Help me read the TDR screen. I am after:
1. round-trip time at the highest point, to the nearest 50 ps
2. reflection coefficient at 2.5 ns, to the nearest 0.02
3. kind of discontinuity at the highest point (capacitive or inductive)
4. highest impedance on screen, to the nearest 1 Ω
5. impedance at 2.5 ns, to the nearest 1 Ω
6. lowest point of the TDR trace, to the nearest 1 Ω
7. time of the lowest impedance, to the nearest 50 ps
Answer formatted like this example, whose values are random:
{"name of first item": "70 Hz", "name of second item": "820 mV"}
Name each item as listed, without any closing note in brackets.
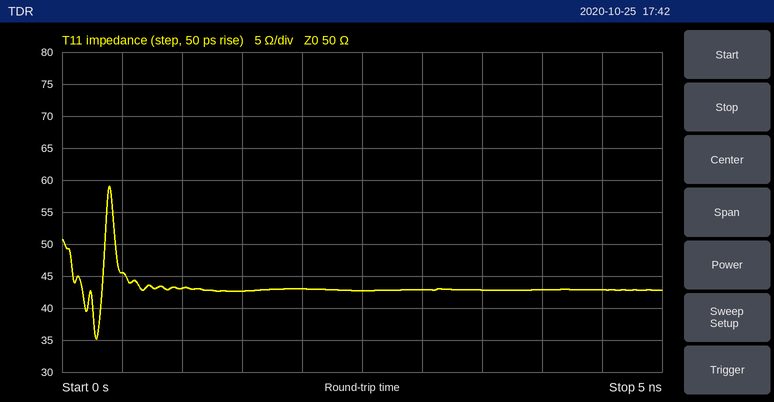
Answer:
{"round-trip time at the highest point, to the nearest 50 ps": "400 ps", "reflection coefficient at 2.5 ns, to the nearest 0.02": "-0.08", "kind of discontinuity at the highest point": "inductive", "highest impedance on screen, to the nearest 1 Ω": "59 Ω", "impedance at 2.5 ns, to the nearest 1 Ω": "43 Ω", "lowest point of the TDR trace, to the nearest 1 Ω": "35 Ω", "time of the lowest impedance, to the nearest 50 ps": "300 ps"}
